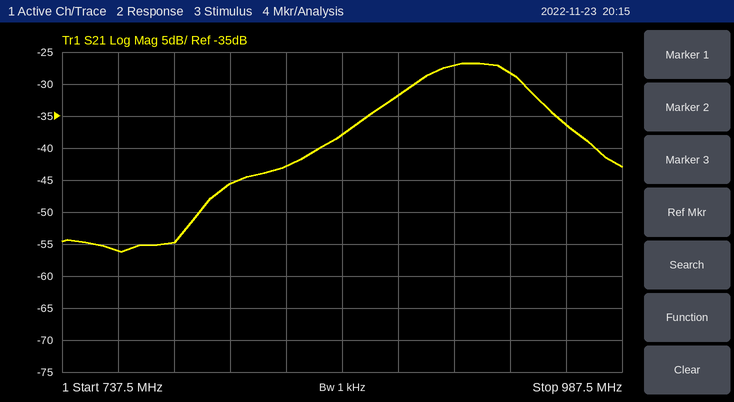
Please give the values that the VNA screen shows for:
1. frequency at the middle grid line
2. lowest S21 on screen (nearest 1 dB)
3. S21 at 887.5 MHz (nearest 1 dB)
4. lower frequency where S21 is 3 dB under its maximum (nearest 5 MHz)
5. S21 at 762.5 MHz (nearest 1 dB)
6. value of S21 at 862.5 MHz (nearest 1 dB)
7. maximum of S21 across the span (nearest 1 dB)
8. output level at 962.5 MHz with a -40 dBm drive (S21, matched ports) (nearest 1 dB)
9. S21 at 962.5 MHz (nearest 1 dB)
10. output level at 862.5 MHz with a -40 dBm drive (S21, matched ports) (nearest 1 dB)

862.5 MHz
-56 dB
-32 dB
895 MHz
-56 dB
-38 dB
-27 dB
-76 dBm
-36 dB
-78 dBm
